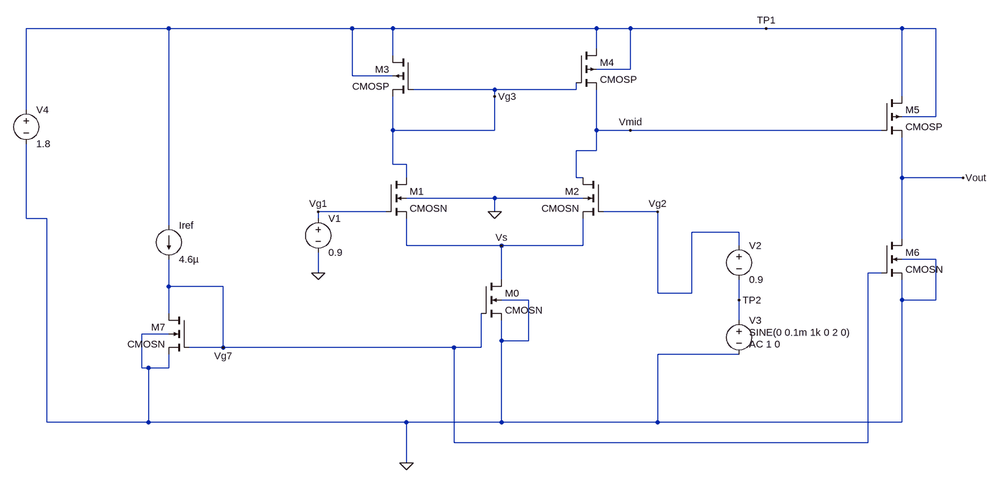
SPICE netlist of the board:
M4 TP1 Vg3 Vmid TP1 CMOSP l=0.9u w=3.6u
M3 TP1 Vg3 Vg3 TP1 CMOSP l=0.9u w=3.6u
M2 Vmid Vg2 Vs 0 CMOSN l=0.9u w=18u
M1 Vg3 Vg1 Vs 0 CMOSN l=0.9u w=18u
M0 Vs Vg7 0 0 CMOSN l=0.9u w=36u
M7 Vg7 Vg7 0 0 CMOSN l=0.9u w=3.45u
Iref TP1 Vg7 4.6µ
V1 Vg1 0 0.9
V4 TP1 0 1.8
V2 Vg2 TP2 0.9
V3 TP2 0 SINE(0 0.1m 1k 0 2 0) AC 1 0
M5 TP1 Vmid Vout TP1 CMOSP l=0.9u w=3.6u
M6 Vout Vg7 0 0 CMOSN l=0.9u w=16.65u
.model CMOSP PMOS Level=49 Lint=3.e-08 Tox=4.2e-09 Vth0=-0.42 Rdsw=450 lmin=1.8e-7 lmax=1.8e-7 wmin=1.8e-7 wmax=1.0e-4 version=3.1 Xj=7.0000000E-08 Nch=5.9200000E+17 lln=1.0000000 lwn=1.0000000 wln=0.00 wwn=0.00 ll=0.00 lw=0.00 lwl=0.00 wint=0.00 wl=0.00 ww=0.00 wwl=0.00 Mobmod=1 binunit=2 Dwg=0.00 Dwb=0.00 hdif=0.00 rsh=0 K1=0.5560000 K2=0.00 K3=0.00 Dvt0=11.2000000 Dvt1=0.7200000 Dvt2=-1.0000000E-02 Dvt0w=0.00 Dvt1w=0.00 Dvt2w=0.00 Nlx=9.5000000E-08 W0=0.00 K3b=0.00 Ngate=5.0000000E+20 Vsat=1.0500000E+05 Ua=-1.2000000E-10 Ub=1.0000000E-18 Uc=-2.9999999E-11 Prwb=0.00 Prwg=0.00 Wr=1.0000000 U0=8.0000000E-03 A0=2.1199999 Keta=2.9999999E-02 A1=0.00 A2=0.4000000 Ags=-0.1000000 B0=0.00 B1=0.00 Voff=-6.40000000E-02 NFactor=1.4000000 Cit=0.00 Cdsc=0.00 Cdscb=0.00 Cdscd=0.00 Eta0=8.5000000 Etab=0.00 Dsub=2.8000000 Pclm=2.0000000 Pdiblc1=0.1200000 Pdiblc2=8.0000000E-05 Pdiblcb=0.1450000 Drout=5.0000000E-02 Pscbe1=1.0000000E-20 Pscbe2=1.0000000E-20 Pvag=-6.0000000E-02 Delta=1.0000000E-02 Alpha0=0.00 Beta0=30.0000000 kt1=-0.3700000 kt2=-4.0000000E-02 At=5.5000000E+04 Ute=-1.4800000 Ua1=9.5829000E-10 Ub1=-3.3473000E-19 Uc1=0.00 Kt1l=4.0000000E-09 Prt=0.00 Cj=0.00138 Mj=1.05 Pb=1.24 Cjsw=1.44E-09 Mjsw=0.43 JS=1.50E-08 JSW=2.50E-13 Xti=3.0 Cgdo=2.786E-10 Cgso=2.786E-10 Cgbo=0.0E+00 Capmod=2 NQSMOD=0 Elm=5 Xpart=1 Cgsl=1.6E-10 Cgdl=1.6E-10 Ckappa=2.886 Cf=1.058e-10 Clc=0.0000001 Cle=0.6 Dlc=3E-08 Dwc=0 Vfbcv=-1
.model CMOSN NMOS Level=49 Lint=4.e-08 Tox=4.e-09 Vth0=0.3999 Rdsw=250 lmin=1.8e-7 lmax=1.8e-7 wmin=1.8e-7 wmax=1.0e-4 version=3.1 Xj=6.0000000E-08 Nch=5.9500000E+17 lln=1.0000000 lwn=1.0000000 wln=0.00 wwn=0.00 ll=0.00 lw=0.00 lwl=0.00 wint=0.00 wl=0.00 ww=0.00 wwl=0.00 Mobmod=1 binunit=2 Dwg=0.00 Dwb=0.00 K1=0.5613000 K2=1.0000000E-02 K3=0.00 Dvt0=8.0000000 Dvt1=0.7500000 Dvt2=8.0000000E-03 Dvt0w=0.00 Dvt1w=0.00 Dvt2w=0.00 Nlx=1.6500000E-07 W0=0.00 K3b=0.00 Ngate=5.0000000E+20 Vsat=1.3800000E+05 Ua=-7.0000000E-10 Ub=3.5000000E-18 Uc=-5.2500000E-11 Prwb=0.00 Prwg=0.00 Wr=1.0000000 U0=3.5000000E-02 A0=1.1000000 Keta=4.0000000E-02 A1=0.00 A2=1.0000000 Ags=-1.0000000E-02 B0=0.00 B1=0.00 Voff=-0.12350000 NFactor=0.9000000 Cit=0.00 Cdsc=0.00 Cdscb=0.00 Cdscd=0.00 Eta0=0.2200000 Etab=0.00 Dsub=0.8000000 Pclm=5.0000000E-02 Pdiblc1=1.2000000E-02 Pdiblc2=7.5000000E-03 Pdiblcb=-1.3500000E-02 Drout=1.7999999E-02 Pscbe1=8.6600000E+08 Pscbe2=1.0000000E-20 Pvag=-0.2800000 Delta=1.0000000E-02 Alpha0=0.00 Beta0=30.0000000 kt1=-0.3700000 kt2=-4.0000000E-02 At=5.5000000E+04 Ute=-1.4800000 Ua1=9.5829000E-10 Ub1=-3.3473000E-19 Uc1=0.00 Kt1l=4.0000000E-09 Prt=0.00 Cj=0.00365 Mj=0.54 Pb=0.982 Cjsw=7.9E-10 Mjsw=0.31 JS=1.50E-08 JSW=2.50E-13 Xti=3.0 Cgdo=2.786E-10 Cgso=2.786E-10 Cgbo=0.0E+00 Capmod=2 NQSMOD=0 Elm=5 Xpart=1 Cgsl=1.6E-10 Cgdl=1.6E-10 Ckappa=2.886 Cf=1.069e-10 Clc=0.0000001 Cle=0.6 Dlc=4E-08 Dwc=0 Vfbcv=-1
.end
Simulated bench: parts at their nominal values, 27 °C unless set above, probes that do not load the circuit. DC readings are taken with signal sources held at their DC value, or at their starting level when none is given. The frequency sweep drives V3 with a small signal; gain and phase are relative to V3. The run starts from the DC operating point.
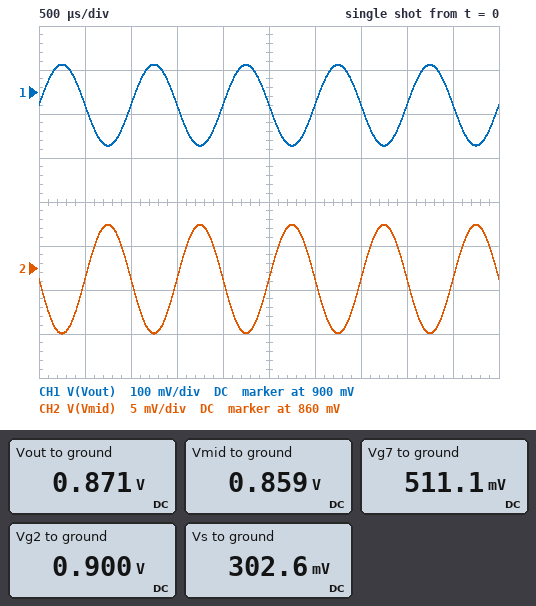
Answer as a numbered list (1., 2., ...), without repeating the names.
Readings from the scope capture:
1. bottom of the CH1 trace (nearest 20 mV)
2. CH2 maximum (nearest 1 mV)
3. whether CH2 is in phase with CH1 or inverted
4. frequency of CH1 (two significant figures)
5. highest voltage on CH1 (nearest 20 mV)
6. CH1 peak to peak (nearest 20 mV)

1. 780 mV
2. 865 mV
3. inverted
4. 1.0 kHz
5. 960 mV
6. 180 mV
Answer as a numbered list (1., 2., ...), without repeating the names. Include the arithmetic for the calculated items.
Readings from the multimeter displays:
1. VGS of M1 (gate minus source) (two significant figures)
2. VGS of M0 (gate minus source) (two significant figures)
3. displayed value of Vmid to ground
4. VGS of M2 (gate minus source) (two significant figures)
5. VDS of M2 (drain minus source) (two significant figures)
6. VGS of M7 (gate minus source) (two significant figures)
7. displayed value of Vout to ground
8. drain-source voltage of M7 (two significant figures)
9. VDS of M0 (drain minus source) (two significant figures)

1. 900 mV - 302.6 mV = 600 mV
2. 511.1 mV = 510 mV
3. 0.859 V
4. 900 mV - 302.6 mV = 600 mV
5. 859 mV - 302.6 mV = 560 mV
6. 511.1 mV = 510 mV
7. 0.871 V
8. 511.1 mV = 510 mV
9. 302.6 mV = 300 mV
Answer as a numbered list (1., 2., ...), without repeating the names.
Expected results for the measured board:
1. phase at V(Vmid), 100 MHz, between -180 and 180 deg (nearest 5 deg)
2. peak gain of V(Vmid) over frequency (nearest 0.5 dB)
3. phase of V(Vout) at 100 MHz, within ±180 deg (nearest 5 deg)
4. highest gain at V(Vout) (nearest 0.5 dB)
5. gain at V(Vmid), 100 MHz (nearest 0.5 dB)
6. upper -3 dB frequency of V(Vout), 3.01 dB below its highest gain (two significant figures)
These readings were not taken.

1. 70 deg
2. 36.0 dB
3. -170 deg
4. 59.5 dB
5. 20.5 dB
6. 9.4 MHz
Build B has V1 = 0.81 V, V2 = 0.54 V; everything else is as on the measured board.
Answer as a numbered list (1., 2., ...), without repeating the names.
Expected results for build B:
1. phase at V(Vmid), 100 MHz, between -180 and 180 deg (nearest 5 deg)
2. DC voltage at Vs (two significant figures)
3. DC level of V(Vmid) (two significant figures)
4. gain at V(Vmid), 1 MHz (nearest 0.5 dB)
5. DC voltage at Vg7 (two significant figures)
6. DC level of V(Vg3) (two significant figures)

1. 120 deg
2. 190 mV
3. 1.8 V
4. -29.0 dB
5. 510 mV
6. 640 mV
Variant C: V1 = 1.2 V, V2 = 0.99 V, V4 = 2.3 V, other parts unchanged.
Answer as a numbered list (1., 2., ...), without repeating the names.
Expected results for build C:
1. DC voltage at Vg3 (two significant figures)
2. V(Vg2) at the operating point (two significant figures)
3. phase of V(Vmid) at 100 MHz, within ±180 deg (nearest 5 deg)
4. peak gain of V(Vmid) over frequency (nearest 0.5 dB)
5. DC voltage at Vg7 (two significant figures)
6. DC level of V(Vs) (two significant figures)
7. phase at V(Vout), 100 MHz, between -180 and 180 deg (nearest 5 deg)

1. 1.1 V
2. 990 mV
3. 150 deg
4. -16.5 dB
5. 510 mV
6. 500 mV
7. -155 deg
